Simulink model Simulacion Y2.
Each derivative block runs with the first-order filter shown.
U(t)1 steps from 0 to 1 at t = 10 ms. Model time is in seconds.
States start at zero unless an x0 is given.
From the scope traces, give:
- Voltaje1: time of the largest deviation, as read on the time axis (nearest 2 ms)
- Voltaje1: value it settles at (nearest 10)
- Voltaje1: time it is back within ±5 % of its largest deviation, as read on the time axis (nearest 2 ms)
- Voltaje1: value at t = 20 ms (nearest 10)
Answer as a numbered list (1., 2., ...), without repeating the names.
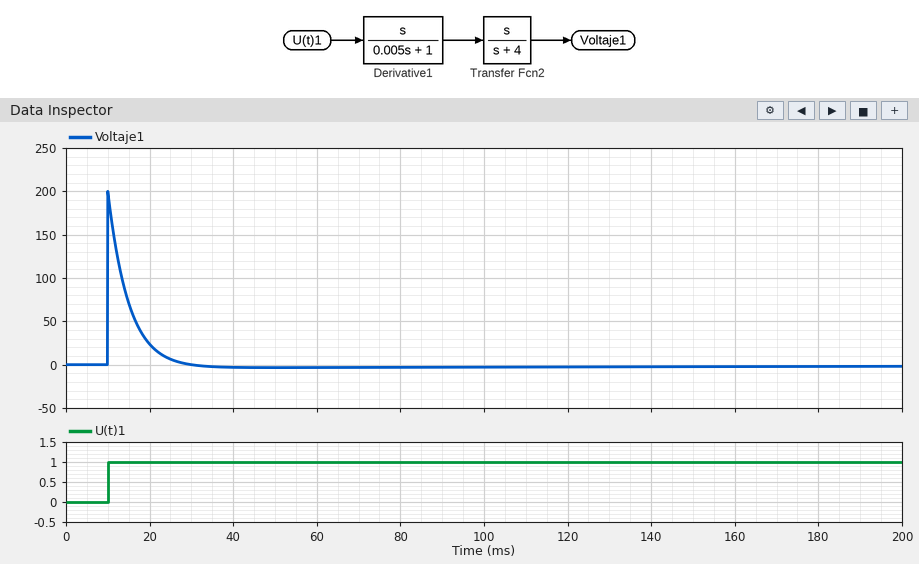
1. 10 ms
2. 0
3. 24 ms
4. 20
